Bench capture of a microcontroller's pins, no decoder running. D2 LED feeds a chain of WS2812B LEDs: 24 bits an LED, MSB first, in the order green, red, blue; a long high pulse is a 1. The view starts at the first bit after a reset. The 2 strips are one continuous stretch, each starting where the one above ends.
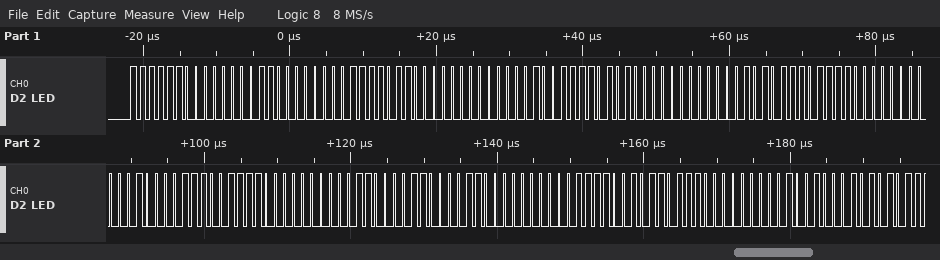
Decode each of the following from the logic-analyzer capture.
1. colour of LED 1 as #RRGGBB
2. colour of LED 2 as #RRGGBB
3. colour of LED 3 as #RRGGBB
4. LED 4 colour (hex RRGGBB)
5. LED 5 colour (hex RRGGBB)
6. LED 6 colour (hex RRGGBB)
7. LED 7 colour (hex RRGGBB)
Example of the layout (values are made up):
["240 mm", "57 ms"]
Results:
["#03FC00", "#00F609", "#00EA15", "#00DE21", "#00CF30", "#00C33C", "#00B748"]
